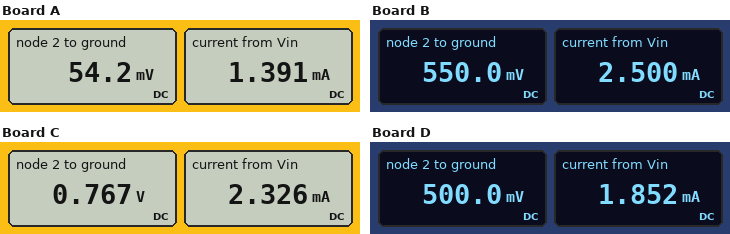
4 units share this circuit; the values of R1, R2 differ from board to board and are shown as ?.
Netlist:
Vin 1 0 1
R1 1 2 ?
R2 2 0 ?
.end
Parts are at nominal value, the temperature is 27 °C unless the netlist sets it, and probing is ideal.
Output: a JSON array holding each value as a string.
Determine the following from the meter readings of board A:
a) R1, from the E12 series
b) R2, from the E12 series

["680 Ω", "39 Ω"]
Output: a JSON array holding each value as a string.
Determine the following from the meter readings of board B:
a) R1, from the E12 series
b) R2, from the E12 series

["180 Ω", "220 Ω"]
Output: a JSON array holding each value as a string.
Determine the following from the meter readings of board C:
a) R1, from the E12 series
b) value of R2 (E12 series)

["100 Ω", "330 Ω"]
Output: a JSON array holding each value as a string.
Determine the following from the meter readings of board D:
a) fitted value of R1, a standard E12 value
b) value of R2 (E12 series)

["270 Ω", "270 Ω"]
